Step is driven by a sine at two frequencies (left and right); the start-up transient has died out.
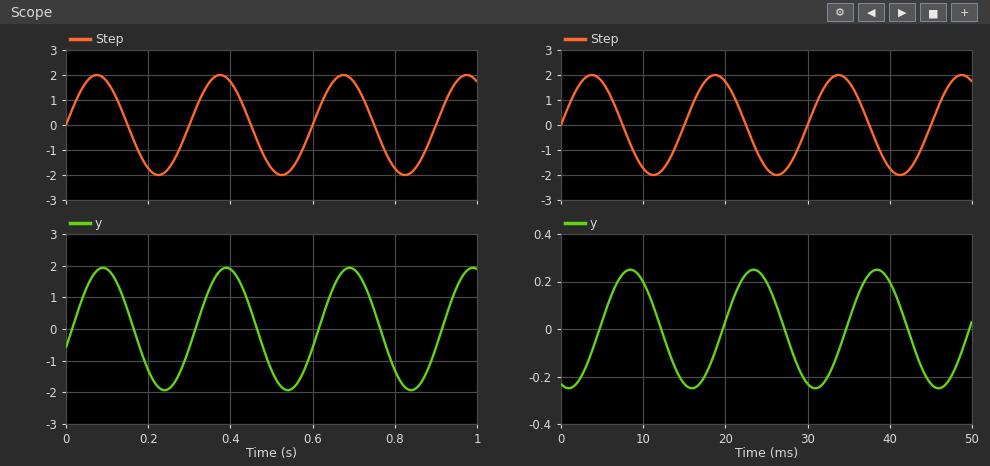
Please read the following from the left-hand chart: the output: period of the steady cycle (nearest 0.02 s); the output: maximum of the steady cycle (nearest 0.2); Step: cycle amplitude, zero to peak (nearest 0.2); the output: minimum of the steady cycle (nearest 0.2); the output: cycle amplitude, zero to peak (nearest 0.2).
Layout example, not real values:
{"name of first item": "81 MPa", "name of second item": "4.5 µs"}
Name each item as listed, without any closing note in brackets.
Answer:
{"the output: period of the steady cycle": "0.30 s", "the output: maximum of the steady cycle": "2.0", "Step: cycle amplitude, zero to peak": "2.0", "the output: minimum of the steady cycle": "-2.0", "the output: cycle amplitude, zero to peak": "2.0"}
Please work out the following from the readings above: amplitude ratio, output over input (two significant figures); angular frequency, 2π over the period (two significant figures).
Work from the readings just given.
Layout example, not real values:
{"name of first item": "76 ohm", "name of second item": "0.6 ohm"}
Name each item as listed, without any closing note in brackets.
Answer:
{"amplitude ratio, output over input": "1.0", "angular frequency, 2π over the period": "21 rad/s"}
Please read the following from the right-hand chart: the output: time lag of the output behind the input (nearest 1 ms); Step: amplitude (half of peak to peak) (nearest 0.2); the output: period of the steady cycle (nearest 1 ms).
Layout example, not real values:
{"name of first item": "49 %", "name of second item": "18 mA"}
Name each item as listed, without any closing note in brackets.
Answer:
{"the output: time lag of the output behind the input": "5 ms", "Step: amplitude (half of peak to peak)": "2.0", "the output: period of the steady cycle": "15 ms"}
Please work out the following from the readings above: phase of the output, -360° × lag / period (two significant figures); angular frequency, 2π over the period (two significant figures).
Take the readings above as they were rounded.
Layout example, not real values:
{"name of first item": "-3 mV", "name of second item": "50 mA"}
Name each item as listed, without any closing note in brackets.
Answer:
{"phase of the output, -360° × lag / period": "-120°", "angular frequency, 2π over the period": "0.42 rad/ms"}
